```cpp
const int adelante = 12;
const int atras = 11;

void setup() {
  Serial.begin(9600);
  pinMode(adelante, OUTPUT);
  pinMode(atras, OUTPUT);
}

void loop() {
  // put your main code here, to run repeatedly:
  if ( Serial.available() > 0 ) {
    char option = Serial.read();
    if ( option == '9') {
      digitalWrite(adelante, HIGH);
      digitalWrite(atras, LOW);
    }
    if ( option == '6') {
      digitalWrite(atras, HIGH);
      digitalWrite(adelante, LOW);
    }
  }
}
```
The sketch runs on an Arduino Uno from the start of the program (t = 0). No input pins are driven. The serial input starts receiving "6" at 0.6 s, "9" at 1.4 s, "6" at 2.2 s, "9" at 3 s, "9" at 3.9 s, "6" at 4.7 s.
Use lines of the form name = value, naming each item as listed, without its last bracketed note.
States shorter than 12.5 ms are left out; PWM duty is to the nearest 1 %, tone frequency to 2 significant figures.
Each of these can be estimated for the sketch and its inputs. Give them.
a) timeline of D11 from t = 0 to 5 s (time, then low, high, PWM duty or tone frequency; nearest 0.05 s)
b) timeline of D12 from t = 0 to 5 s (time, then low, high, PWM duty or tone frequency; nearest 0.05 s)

timeline of D11 from t = 0 to 5 s = 0 s low; 0.6 s high; 1.4 s low; 2.2 s high; 3 s low; 4.7 s high
timeline of D12 from t = 0 to 5 s = 0 s low; 1.4 s high; 2.2 s low; 3 s high; 4.7 s low
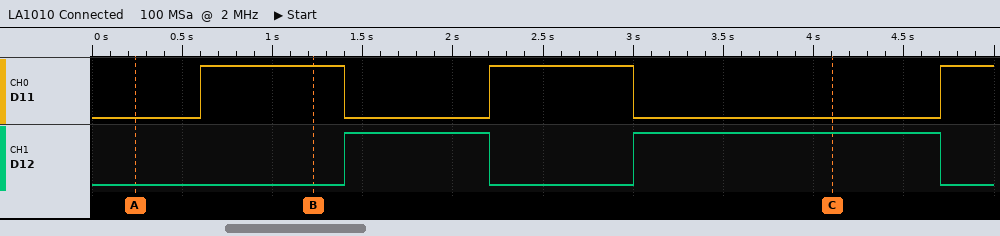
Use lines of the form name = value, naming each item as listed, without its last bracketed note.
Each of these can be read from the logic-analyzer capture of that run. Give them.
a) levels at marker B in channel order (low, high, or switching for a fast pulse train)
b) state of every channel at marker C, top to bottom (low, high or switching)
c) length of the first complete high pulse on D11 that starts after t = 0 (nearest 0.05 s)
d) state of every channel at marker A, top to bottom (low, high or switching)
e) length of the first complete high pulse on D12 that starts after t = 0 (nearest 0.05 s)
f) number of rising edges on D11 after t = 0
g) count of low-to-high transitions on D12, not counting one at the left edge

levels at marker B in channel order = D11 high, D12 low
state of every channel at marker C, top to bottom = D11 low, D12 high
length of the first complete high pulse on D11 that starts after t = 0 = 0.80 s
state of every channel at marker A, top to bottom = D11 low, D12 low
length of the first complete high pulse on D12 that starts after t = 0 = 0.80 s
number of rising edges on D11 after t = 0 = 3
count of low-to-high transitions on D12, not counting one at the left edge = 2
